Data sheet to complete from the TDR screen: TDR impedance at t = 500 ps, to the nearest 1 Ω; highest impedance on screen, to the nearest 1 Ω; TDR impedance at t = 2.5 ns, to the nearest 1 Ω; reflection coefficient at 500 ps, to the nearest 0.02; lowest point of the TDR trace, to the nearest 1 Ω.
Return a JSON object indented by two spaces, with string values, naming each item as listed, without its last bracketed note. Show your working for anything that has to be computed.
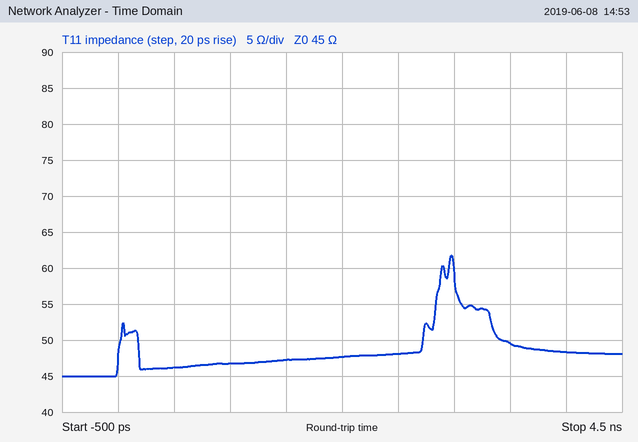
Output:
{
  "TDR impedance at t = 500 ps, to the nearest 1 Ω": "46 Ω",
  "highest impedance on screen, to the nearest 1 Ω": "62 Ω",
  "TDR impedance at t = 2.5 ns, to the nearest 1 Ω": "48 Ω",
  "reflection coefficient at 500 ps, to the nearest 0.02": "(46 − 45)/(46 + 45) ≈ +0.0110, so +0.02 to the nearest 0.02",
  "lowest point of the TDR trace, to the nearest 1 Ω": "45 Ω"
}
